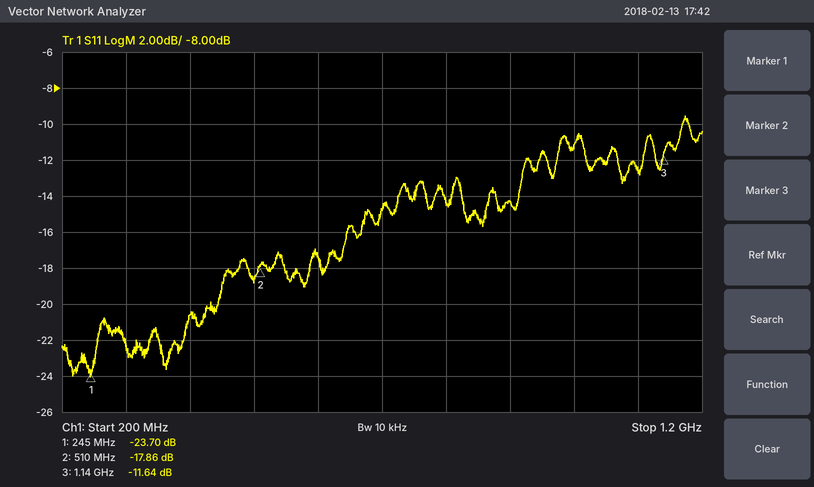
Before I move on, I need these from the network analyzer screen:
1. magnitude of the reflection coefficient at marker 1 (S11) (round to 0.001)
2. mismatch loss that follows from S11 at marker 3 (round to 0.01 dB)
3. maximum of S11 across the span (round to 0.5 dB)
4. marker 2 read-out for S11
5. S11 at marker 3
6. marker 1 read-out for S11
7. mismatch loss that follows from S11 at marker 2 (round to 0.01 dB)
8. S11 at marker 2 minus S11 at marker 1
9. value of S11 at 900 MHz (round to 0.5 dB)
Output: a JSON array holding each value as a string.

["0.065", "0.31 dB", "-9.5 dB", "-17.86 dB", "-11.64 dB", "-23.70 dB", "0.07 dB", "5.84 dB", "-14.5 dB"]
